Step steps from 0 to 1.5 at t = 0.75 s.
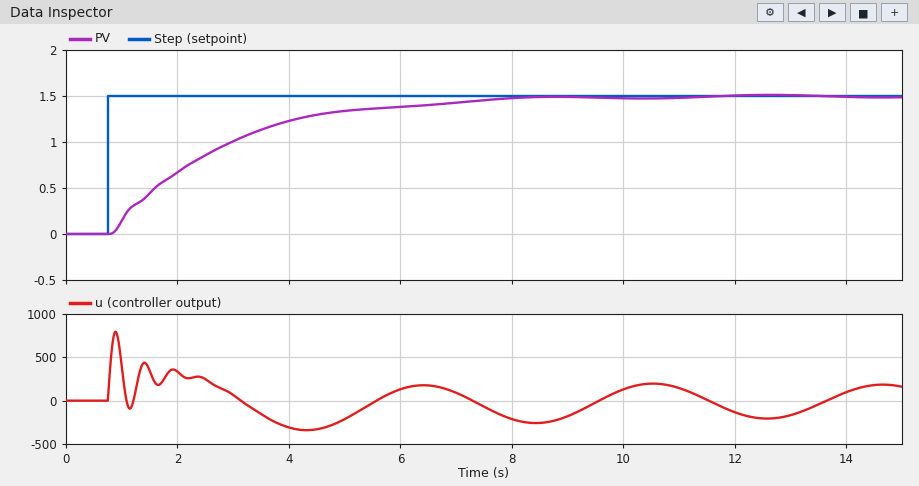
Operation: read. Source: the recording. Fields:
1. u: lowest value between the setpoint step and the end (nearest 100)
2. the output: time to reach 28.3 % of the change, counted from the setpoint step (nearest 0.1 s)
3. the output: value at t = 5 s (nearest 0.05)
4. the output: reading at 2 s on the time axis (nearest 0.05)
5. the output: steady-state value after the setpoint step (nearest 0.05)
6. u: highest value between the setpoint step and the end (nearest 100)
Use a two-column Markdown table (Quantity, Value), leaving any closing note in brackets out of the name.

| Quantity | Value |
|---|---|
| u: lowest value between the setpoint step and the end | -300 |
| the output: time to reach 28.3 % of the change, counted from the setpoint step | 0.7 s |
| the output: value at t = 5 s | 1.35 |
| the output: reading at 2 s on the time axis | 0.65 |
| the output: steady-state value after the setpoint step | 1.50 |
| u: highest value between the setpoint step and the end | 800 |
